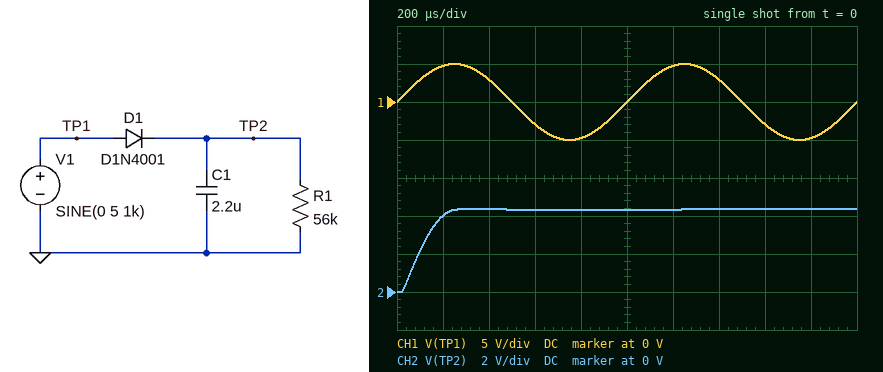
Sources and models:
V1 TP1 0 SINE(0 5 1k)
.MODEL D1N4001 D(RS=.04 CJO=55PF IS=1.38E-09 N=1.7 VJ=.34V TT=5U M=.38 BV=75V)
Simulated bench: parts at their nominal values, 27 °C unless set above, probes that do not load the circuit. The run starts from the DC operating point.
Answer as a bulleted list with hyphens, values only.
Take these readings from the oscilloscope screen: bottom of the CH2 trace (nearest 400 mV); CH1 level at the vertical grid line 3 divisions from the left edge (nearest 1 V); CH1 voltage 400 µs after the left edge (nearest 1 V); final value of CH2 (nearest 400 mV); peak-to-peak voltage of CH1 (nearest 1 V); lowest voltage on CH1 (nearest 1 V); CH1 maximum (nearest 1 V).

- 0 V
- -3 V
- 3 V
- 4.4 V
- 10 V
- -5 V
- 5 V
